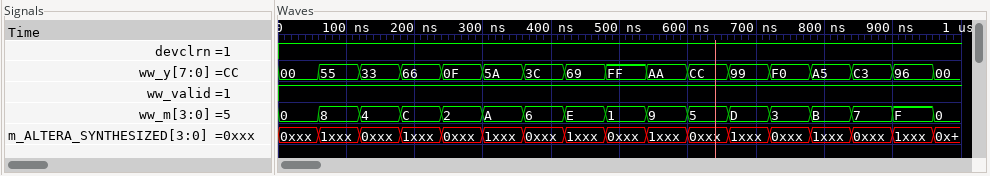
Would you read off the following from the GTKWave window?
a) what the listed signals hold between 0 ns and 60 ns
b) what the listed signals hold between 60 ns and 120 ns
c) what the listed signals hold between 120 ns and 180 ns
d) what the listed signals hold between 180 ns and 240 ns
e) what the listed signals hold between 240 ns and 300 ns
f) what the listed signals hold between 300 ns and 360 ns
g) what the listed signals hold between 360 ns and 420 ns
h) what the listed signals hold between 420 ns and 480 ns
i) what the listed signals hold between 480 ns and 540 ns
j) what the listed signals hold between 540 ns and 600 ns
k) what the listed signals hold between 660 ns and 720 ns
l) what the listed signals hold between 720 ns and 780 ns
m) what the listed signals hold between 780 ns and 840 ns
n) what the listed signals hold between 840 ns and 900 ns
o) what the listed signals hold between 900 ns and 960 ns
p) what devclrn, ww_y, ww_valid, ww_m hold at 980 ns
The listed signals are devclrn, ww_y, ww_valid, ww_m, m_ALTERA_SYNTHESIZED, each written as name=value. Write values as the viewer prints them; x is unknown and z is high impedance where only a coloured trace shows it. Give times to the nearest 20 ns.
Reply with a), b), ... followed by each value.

a) devclrn=1, ww_y=00, ww_valid=1, ww_m=0, m_ALTERA_SYNTHESIZED=0xxx
b) devclrn=1, ww_y=55, ww_valid=1, ww_m=8, m_ALTERA_SYNTHESIZED=1xxx
c) devclrn=1, ww_y=33, ww_valid=1, ww_m=4, m_ALTERA_SYNTHESIZED=0xxx
d) devclrn=1, ww_y=66, ww_valid=1, ww_m=C, m_ALTERA_SYNTHESIZED=1xxx
e) devclrn=1, ww_y=0F, ww_valid=1, ww_m=2, m_ALTERA_SYNTHESIZED=0xxx
f) devclrn=1, ww_y=5A, ww_valid=1, ww_m=A, m_ALTERA_SYNTHESIZED=1xxx
g) devclrn=1, ww_y=3C, ww_valid=1, ww_m=6, m_ALTERA_SYNTHESIZED=0xxx
h) devclrn=1, ww_y=69, ww_valid=1, ww_m=E, m_ALTERA_SYNTHESIZED=1xxx
i) devclrn=1, ww_y=FF, ww_valid=1, ww_m=1, m_ALTERA_SYNTHESIZED=0xxx
j) devclrn=1, ww_y=AA, ww_valid=1, ww_m=9, m_ALTERA_SYNTHESIZED=1xxx
k) devclrn=1, ww_y=99, ww_valid=1, ww_m=D, m_ALTERA_SYNTHESIZED=1xxx
l) devclrn=1, ww_y=F0, ww_valid=1, ww_m=3, m_ALTERA_SYNTHESIZED=0xxx
m) devclrn=1, ww_y=A5, ww_valid=1, ww_m=B, m_ALTERA_SYNTHESIZED=1xxx
n) devclrn=1, ww_y=C3, ww_valid=1, ww_m=7, m_ALTERA_SYNTHESIZED=0xxx
o) devclrn=1, ww_y=96, ww_valid=1, ww_m=F, m_ALTERA_SYNTHESIZED=1xxx
p) devclrn=1, ww_y=00, ww_valid=1, ww_m=0
